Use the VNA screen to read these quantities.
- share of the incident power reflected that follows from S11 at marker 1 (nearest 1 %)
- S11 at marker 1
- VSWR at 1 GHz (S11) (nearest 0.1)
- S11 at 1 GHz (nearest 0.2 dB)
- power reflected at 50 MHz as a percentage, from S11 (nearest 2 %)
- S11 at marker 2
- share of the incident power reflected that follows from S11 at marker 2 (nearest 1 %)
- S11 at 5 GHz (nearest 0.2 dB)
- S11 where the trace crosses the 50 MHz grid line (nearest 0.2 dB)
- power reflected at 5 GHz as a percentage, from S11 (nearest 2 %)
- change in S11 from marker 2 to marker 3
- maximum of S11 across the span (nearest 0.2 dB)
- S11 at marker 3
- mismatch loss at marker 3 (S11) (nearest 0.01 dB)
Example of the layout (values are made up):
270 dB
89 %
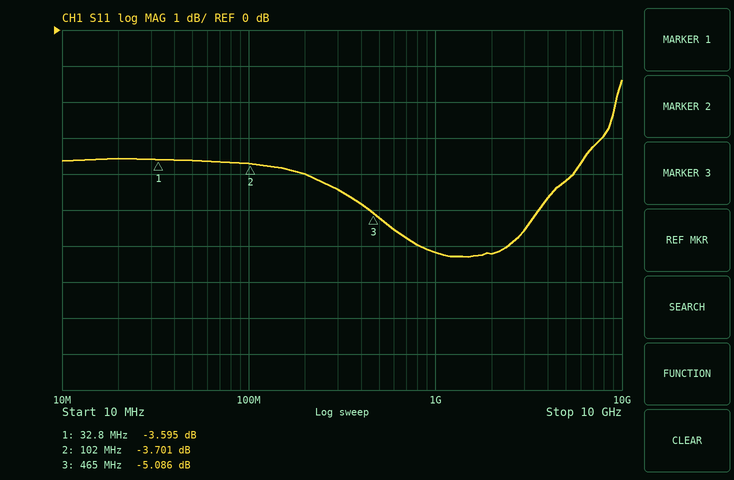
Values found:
44 %
-3.595 dB
2.9
-6.2 dB
44 %
-3.701 dB
43 %
-4.2 dB
-3.6 dB
38 %
-1.385 dB
-1.4 dB
-5.086 dB
1.61 dB
